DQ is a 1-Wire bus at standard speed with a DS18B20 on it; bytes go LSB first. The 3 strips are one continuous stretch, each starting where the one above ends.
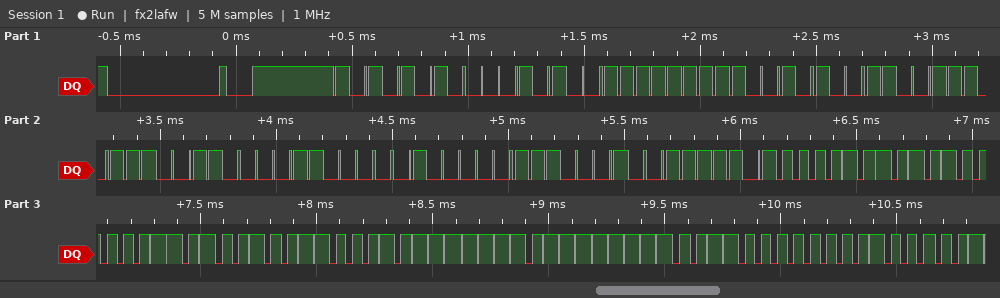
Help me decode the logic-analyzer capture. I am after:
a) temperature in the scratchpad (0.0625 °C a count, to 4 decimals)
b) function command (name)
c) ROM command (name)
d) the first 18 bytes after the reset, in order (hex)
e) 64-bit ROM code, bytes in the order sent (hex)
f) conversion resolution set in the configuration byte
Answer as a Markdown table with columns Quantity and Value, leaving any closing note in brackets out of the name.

| Quantity | Value |
|---|---|
| temperature in the scratchpad | 85.0000 °C |
| function command | Read Scratchpad |
| ROM command | Match ROM |
| the first 18 bytes after the reset, in order | 55 28 FF 29 73 67 18 04 47 BE 50 05 4B 46 7F FF 0C 10 |
| 64-bit ROM code, bytes in the order sent | 28 FF 29 73 67 18 04 47 |
| conversion resolution set in the configuration byte | 12 bits |
